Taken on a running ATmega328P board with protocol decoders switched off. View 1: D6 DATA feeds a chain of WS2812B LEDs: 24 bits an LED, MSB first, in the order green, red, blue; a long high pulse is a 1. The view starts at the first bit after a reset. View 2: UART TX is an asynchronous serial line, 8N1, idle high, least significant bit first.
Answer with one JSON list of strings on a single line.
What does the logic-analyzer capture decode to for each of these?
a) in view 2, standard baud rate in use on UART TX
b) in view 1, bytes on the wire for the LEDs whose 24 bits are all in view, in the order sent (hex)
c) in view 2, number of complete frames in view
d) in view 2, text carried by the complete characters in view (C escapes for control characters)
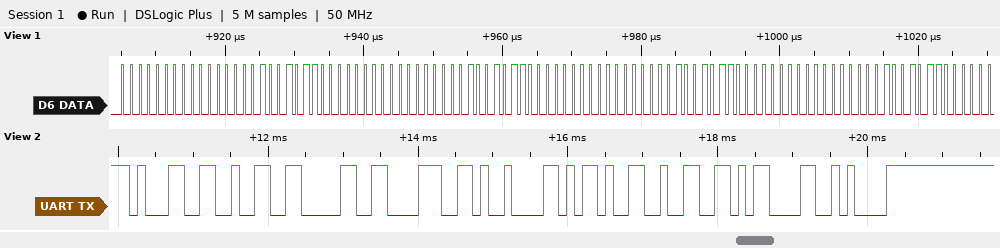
["9600 baud", "00 00 96 00 00 96 00 00 96 00 00 96", "9", "\"1208\\t-2\\r\\n\""]
